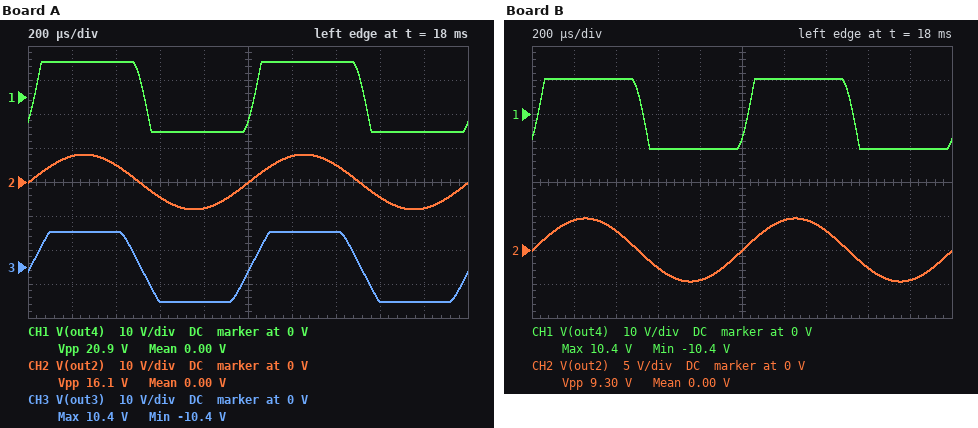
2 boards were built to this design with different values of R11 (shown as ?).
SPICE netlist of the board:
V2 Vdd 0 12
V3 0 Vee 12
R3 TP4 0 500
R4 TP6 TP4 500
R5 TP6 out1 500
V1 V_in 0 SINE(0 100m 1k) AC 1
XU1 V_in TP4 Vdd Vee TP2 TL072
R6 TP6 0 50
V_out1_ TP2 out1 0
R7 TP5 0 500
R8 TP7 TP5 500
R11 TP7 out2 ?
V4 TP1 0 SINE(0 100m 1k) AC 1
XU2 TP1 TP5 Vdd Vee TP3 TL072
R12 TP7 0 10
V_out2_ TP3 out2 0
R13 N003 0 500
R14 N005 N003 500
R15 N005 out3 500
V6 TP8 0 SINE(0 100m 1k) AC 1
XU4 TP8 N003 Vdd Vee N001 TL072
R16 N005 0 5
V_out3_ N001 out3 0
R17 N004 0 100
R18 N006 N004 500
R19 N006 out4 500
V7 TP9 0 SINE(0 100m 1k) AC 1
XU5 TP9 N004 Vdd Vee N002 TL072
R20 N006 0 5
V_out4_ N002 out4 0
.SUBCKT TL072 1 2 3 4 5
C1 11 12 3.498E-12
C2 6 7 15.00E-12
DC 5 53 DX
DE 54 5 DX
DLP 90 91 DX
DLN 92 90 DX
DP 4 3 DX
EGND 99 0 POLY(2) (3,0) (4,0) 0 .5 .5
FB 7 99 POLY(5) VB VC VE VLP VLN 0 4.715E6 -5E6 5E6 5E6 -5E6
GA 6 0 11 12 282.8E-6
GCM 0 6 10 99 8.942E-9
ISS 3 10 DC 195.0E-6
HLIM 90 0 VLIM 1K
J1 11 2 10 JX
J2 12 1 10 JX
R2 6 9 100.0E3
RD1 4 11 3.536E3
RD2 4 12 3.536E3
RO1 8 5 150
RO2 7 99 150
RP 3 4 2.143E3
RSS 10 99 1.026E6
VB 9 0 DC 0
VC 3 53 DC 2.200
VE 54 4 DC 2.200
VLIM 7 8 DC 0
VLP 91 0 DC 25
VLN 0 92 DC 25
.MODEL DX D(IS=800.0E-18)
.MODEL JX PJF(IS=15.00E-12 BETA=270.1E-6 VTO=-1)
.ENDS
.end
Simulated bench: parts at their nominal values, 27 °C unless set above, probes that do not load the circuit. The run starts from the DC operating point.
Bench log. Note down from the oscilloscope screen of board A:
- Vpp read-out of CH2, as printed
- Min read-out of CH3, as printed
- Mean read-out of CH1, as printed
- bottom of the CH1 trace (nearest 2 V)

16.1 V
-10.4 V
0.00 V
-10 V
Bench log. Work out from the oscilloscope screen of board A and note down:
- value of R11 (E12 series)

390 Ω
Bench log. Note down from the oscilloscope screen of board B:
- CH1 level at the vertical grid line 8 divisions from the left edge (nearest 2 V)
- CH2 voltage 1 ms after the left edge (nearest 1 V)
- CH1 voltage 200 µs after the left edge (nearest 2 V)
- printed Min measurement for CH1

-10 V
0 V
10 V
-10.4 V
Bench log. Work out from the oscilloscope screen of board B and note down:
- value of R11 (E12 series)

220 Ω
